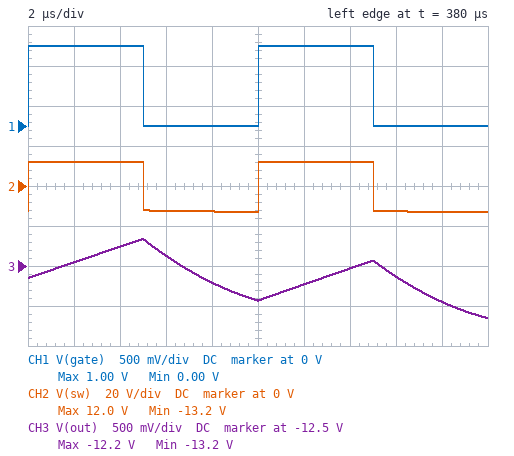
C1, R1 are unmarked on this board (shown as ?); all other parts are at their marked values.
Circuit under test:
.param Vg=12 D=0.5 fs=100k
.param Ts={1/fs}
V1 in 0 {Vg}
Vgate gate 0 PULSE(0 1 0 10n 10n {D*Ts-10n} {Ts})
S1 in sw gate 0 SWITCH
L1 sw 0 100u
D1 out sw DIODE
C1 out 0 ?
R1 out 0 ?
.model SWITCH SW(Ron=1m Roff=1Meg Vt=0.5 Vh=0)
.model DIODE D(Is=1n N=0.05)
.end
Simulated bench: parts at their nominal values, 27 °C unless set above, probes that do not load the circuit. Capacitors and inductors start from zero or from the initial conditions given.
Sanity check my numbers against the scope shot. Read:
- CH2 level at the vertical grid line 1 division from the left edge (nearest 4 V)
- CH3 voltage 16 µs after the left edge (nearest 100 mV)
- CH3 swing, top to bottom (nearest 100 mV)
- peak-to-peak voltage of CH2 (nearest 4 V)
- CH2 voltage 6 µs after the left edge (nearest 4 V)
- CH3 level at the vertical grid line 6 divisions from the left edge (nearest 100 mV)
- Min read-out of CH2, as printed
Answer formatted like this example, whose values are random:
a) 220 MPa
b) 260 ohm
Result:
a) 12 V
b) -12.6 V
c) 1.0 V
d) 24 V
e) -12 V
f) -12.7 V
g) -13.2 V
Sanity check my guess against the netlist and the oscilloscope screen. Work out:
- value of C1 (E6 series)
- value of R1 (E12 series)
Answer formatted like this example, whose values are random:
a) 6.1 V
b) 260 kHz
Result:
a) 4.7 µF
b) 27 Ω
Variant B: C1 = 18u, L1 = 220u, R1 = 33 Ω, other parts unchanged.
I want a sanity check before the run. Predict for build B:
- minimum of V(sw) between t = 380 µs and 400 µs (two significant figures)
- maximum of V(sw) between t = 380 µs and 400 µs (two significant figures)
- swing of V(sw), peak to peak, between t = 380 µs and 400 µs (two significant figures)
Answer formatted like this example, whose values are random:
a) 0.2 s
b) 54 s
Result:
a) -21 V
b) 12 V
c) 33 V
